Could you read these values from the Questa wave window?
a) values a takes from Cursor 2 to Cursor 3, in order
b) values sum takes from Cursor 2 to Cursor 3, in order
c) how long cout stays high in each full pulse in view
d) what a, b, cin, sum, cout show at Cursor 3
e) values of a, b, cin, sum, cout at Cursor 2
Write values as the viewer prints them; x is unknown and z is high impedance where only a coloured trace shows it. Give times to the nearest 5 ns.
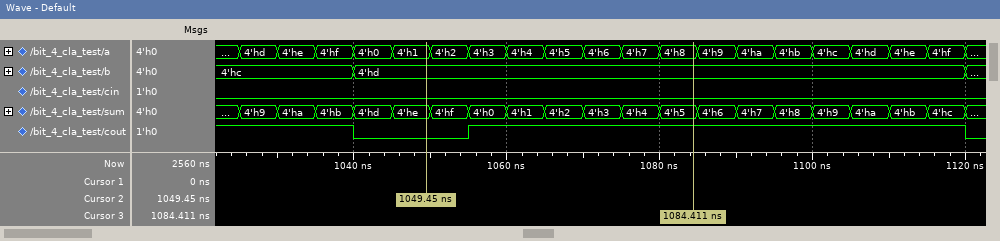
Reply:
4'h1, 4'h2, 4'h3, 4'h4, 4'h5, 4'h6, 4'h7, 4'h8
4'he, 4'hf, 4'h0, 4'h1, 4'h2, 4'h3, 4'h4, 4'h5
65 ns
a=4'h8, b=4'hd, cin=0, sum=4'h5, cout=1
a=4'h1, b=4'hd, cin=0, sum=4'he, cout=0
